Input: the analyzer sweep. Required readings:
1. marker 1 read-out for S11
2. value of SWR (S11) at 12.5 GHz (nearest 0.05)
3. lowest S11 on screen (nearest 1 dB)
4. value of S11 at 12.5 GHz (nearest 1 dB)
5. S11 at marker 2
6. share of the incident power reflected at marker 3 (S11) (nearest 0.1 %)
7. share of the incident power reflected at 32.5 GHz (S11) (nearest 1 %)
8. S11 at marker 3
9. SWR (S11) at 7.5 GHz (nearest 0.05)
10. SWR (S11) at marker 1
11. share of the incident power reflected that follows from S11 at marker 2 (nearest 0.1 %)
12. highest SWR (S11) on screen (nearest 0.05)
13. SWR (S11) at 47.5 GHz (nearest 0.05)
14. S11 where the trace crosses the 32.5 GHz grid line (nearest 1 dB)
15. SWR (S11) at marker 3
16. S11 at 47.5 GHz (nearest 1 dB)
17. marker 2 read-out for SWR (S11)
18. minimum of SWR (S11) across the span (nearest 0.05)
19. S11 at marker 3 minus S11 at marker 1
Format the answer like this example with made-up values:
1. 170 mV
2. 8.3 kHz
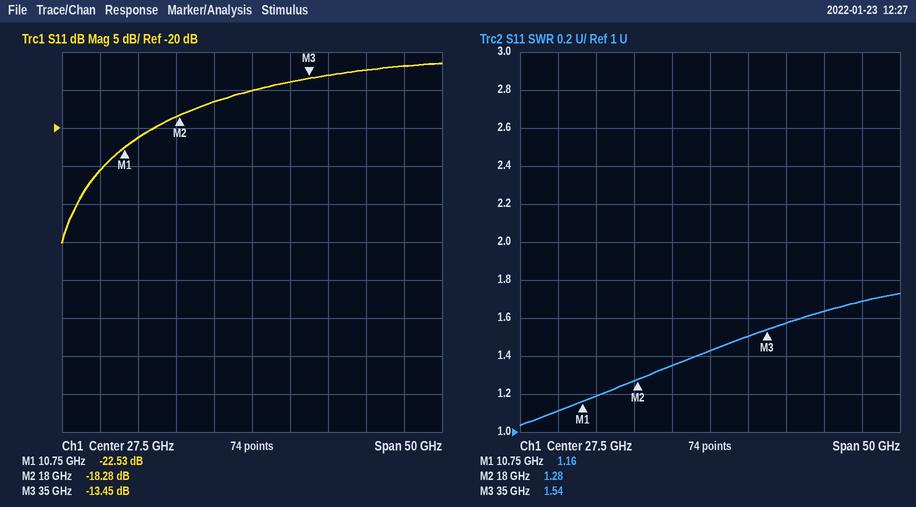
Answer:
1. -22.53 dB
2. 1.20
3. -35 dB
4. -21 dB
5. -18.28 dB
6. 4.5 %
7. 4 %
8. -13.45 dB
9. 1.10
10. 1.16
11. 1.5 %
12. 1.75
13. 1.70
14. -14 dB
15. 1.54
16. -12 dB
17. 1.28
18. 1.05
19. 9.08 dB
